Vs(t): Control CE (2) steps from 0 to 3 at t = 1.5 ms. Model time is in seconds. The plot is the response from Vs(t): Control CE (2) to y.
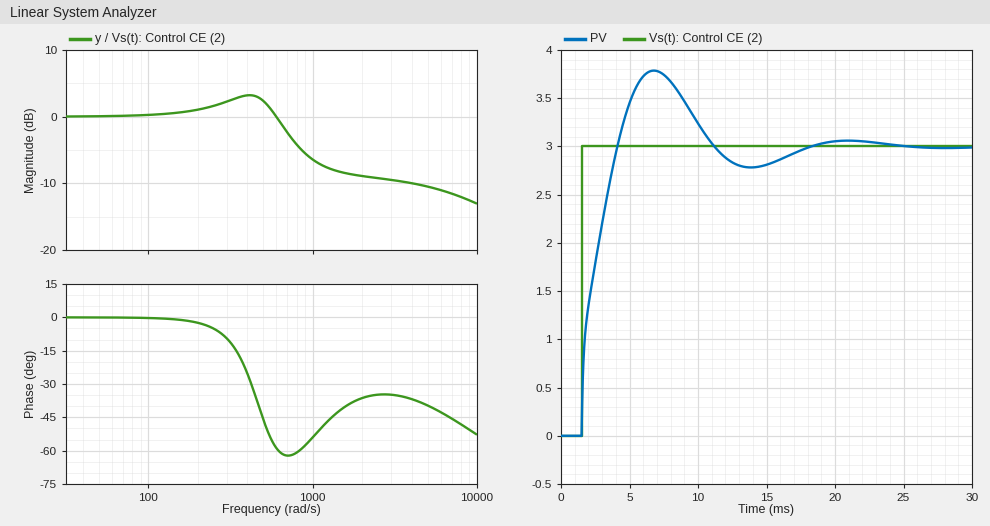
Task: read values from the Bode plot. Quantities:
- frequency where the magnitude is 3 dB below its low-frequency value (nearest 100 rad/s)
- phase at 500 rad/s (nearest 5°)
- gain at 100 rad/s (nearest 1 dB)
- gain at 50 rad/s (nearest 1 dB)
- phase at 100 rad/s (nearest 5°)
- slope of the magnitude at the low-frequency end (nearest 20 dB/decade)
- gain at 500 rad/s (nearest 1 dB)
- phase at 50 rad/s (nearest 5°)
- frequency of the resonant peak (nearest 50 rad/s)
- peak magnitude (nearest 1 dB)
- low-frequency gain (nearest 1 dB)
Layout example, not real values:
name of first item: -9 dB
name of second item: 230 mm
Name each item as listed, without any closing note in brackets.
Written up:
frequency where the magnitude is 3 dB below its low-frequency value: 700 rad/s
phase at 500 rad/s: -45°
gain at 100 rad/s: 0 dB
gain at 50 rad/s: 0 dB
phase at 100 rad/s: 0°
slope of the magnitude at the low-frequency end: 0 dB/decade
gain at 500 rad/s: 2 dB
phase at 50 rad/s: 0°
frequency of the resonant peak: 400 rad/s
peak magnitude: 3 dB
low-frequency gain: 0 dB
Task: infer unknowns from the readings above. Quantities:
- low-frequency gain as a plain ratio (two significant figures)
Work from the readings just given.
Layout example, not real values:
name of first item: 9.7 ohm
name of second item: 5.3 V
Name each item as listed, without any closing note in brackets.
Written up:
low-frequency gain as a plain ratio: 1.0
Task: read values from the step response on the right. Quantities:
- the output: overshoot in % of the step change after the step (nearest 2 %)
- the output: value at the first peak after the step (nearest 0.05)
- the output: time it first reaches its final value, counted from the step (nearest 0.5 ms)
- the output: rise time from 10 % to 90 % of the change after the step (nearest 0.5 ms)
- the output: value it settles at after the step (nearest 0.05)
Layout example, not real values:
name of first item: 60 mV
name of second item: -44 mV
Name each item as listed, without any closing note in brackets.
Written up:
the output: overshoot in % of the step change after the step: 26 %
the output: value at the first peak after the step: 3.80
the output: time it first reaches its final value, counted from the step: 2.5 ms
the output: rise time from 10 % to 90 % of the change after the step: 2.0 ms
the output: value it settles at after the step: 3.00
